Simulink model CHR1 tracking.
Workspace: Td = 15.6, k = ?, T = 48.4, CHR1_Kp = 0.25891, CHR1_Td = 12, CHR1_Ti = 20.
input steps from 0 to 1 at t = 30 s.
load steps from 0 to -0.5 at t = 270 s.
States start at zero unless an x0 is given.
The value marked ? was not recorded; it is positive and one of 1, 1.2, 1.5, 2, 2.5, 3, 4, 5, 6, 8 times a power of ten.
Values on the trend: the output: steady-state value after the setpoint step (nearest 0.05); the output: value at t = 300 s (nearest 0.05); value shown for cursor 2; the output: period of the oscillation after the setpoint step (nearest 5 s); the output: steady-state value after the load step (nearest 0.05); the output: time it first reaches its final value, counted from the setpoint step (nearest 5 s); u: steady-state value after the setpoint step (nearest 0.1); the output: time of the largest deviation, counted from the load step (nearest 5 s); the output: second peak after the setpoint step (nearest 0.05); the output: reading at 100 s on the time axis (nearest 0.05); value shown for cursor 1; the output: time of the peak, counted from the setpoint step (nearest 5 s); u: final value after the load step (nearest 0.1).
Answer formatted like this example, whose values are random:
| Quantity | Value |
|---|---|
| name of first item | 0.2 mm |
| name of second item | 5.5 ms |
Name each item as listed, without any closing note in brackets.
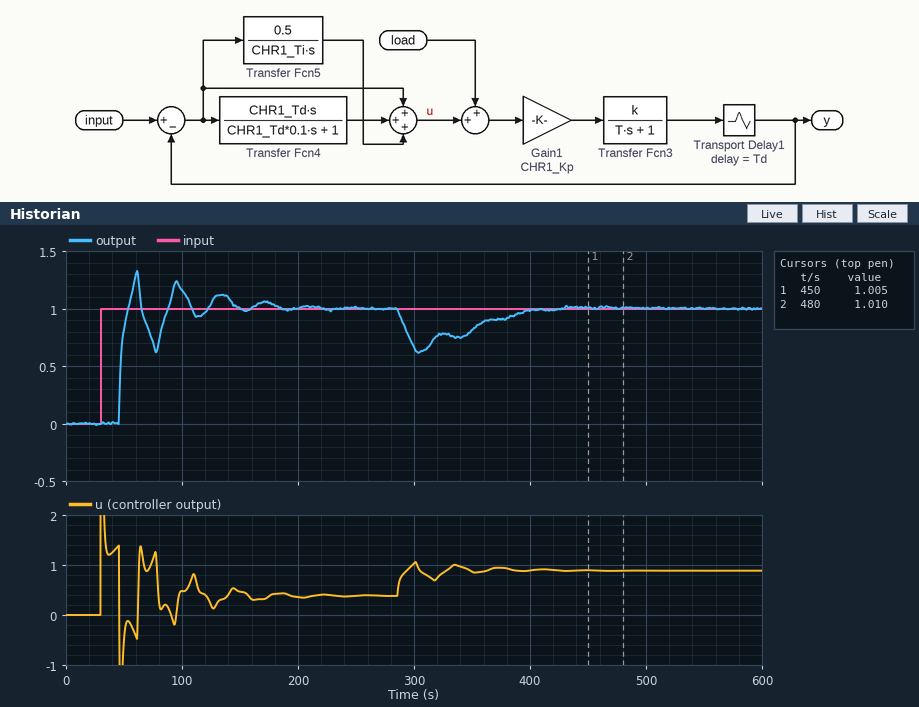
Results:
| Quantity | Value |
|---|---|
| the output: steady-state value after the setpoint step | 1.00 |
| the output: value at t = 300 s | 0.65 |
| value shown for cursor 2 | 1.010 |
| the output: period of the oscillation after the setpoint step | 35 s |
| the output: steady-state value after the load step | 1.00 |
| the output: time it first reaches its final value, counted from the setpoint step | 25 s |
| u: steady-state value after the setpoint step | 0.4 |
| the output: time of the largest deviation, counted from the load step | 35 s |
| the output: second peak after the setpoint step | 1.25 |
| the output: reading at 100 s on the time axis | 1.15 |
| value shown for cursor 1 | 1.005 |
| the output: time of the peak, counted from the setpoint step | 30 s |
| u: final value after the load step | 0.9 |
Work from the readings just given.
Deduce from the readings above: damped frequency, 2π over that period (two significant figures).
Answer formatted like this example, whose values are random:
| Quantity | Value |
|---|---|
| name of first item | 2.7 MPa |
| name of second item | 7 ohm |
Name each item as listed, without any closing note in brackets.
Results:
| Quantity | Value |
|---|---|
| damped frequency, 2π over that period | 0.18 rad/s |
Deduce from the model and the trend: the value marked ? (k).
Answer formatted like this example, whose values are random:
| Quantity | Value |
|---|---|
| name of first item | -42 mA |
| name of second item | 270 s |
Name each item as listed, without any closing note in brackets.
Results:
| Quantity | Value |
|---|---|
| the value marked ? | 10 |
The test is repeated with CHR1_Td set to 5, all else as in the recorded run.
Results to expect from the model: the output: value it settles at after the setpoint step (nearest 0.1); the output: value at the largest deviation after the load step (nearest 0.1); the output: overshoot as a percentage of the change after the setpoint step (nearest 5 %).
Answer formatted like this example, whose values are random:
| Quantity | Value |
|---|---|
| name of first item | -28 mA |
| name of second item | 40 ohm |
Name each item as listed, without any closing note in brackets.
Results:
| Quantity | Value |
|---|---|
| the output: value it settles at after the setpoint step | 1.0 |
| the output: value at the largest deviation after the load step | 0.6 |
| the output: overshoot as a percentage of the change after the setpoint step | 15 % |
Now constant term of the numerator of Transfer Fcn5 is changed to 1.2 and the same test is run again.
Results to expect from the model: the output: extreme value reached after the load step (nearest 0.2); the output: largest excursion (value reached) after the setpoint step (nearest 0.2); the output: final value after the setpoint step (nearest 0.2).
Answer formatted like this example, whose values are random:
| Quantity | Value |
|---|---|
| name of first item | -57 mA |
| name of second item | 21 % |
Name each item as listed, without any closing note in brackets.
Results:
| Quantity | Value |
|---|---|
| the output: extreme value reached after the load step | 0.6 |
| the output: largest excursion (value reached) after the setpoint step | 1.6 |
| the output: final value after the setpoint step | 1.0 |
